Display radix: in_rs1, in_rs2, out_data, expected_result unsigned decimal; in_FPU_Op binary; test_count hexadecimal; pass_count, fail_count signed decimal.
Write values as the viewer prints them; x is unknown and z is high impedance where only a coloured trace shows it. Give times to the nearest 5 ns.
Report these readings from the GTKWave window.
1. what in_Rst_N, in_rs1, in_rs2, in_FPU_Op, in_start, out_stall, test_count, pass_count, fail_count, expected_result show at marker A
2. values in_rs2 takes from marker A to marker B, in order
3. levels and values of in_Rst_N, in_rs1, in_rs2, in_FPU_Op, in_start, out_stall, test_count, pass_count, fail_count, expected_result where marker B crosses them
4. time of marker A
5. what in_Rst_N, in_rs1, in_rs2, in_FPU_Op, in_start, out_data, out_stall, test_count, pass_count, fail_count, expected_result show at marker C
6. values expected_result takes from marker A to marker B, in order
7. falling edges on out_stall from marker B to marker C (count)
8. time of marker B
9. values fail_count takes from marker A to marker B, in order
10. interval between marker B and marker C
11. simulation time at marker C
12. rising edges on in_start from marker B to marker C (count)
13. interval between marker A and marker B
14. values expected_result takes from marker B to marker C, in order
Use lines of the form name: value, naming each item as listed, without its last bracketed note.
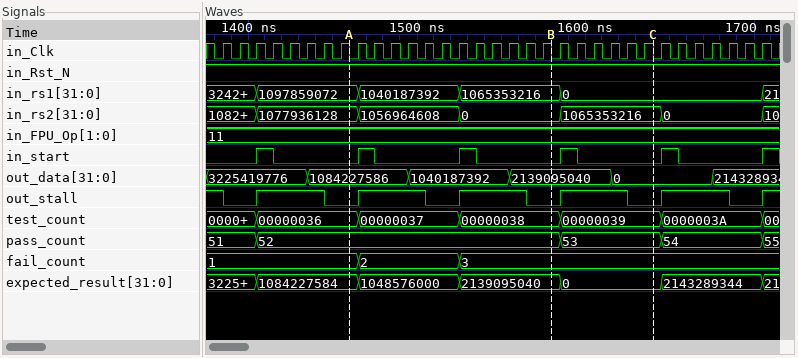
what in_Rst_N, in_rs1, in_rs2, in_FPU_Op, in_start, out_stall, test_count, pass_count, fail_count, expected_result show at marker A: in_Rst_N=1, in_rs1=1097859072, in_rs2=1077936128, in_FPU_Op=11, in_start=0, out_stall=0, test_count=00000036, pass_count=52, fail_count=1, expected_result=1084227584
values in_rs2 takes from marker A to marker B, in order: 1077936128, 1056964608, 0
levels and values of in_Rst_N, in_rs1, in_rs2, in_FPU_Op, in_start, out_stall, test_count, pass_count, fail_count, expected_result where marker B crosses them: in_Rst_N=1, in_rs1=1065353216, in_rs2=0, in_FPU_Op=11, in_start=0, out_stall=0, test_count=00000038, pass_count=52, fail_count=3, expected_result=2139095040
time of marker A: 1460 ns
what in_Rst_N, in_rs1, in_rs2, in_FPU_Op, in_start, out_data, out_stall, test_count, pass_count, fail_count, expected_result show at marker C: in_Rst_N=1, in_rs1=0, in_rs2=1065353216, in_FPU_Op=11, in_start=0, out_data=0, out_stall=0, test_count=00000039, pass_count=53, fail_count=3, expected_result=0
values expected_result takes from marker A to marker B, in order: 1084227584, 1048576000, 2139095040
falling edges on out_stall from marker B to marker C: 1
time of marker B: 1580 ns
values fail_count takes from marker A to marker B, in order: 1, 2, 3
interval between marker B and marker C: 60 ns
simulation time at marker C: 1640 ns
rising edges on in_start from marker B to marker C: 1
interval between marker A and marker B: 120 ns
values expected_result takes from marker B to marker C, in order: 2139095040, 0
